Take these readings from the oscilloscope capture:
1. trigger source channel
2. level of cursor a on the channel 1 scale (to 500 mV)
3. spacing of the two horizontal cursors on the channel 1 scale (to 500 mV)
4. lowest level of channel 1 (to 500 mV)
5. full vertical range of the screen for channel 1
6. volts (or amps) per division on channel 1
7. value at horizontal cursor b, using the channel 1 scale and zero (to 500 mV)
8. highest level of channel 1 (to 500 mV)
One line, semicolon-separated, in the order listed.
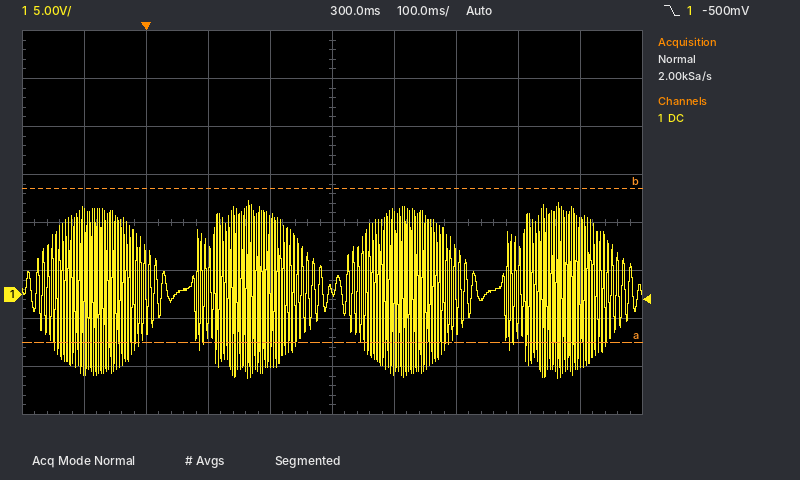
channel 1; -5.0 V; 16.0 V; -9.0 V; 40 V; 5 V; 11.0 V; 10.0 V
